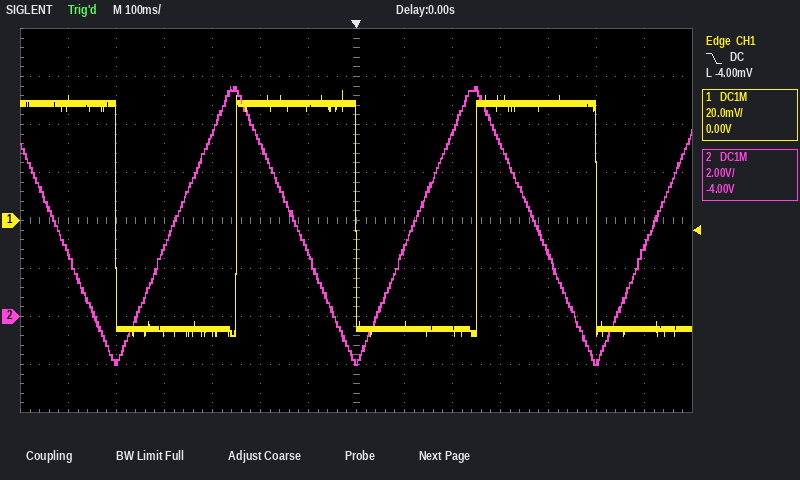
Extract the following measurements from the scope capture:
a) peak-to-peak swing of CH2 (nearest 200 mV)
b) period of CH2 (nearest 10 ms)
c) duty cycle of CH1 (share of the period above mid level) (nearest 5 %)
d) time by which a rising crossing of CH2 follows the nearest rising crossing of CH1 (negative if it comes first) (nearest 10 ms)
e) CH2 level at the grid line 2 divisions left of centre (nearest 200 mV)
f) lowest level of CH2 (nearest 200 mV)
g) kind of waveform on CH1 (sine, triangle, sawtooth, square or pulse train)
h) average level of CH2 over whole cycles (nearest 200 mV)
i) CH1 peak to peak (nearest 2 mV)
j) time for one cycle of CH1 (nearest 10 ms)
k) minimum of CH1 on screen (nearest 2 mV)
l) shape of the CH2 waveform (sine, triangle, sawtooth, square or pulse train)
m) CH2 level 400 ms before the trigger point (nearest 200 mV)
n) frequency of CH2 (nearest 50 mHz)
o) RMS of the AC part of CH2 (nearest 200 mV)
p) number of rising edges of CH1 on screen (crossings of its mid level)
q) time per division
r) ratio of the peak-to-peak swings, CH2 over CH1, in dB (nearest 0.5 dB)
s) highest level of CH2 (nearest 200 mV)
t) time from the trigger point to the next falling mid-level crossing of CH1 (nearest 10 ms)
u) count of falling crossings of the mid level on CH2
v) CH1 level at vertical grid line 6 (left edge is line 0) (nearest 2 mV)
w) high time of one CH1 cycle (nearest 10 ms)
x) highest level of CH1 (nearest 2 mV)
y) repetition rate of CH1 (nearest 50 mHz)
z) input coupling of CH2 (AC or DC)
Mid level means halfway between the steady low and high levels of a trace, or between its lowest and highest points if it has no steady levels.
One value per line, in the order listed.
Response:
11.6 V
500 ms
50 %
-130 ms
7.2 V
-2.0 V
square
3.8 V
102 mV
500 ms
-48 mV
triangle
2.8 V
2.00 Hz
3.4 V
2
100 ms
41.0 dB
9.6 V
500 ms
3
48 mV
250 ms
54 mV
2.00 Hz
DC
